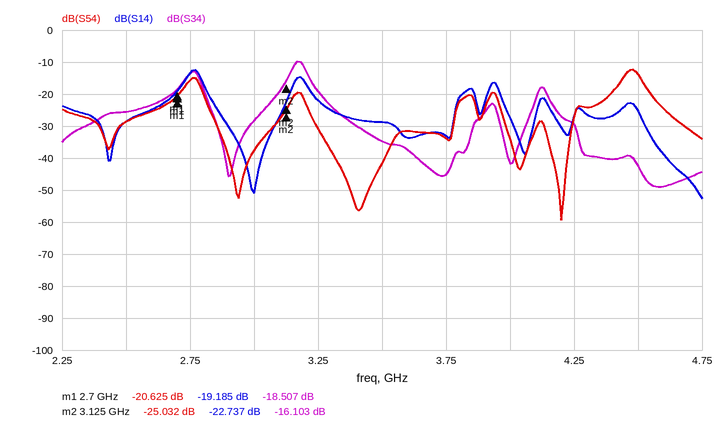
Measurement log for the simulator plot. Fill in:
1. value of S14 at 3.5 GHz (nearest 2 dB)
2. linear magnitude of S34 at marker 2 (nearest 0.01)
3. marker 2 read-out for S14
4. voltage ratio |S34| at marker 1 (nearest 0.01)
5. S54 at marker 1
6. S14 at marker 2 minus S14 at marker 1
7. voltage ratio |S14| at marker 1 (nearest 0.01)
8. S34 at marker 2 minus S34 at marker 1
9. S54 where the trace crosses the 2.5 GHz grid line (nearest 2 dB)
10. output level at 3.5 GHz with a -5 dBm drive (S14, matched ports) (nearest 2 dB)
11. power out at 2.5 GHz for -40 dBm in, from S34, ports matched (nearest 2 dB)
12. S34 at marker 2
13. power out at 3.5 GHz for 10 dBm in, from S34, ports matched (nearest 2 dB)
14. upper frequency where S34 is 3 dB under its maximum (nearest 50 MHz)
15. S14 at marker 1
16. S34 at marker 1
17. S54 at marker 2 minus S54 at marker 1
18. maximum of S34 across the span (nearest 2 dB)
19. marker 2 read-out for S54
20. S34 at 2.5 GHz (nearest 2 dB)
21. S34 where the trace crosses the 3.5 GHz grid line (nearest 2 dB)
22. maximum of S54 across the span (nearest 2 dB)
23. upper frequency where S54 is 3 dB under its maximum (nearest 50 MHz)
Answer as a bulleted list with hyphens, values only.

- -28 dB
- 0.16
- -22.737 dB
- 0.12
- -20.625 dB
- -3.552 dB
- 0.11
- 2.404 dB
- -28 dB
- -34 dBm
- -66 dBm
- -16.103 dB
- -24 dBm
- 3.20 GHz
- -19.185 dB
- -18.507 dB
- -4.407 dB
- -10 dB
- -25.032 dB
- -26 dB
- -34 dB
- -12 dB
- 4.50 GHz
